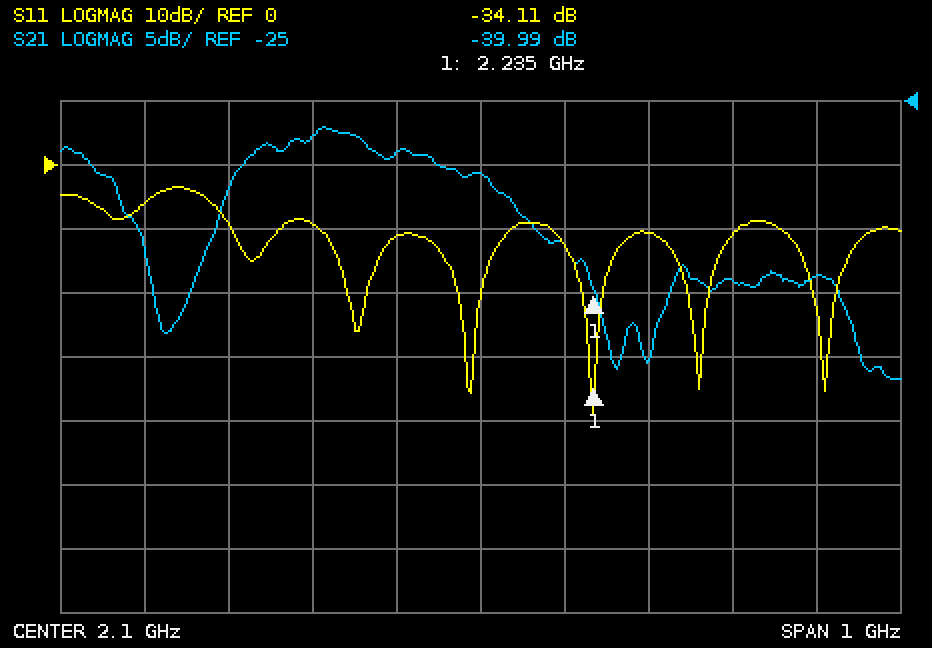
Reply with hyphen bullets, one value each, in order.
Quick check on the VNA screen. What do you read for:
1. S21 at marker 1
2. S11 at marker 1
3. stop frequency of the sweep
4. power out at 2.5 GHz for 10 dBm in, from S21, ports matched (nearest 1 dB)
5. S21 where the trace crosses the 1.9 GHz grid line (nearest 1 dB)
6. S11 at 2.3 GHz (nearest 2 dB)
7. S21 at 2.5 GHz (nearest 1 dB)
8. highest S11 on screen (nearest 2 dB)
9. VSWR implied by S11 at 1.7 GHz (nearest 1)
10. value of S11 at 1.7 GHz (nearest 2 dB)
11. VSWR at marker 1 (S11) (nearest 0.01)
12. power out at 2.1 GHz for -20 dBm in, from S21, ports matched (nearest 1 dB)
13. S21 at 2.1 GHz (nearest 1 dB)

- -39.99 dB
- -34.11 dB
- 2.6 GHz
- -29 dBm
- -28 dB
- -10 dB
- -39 dB
- -4 dB
- 3
- -6 dB
- 1.04
- -51 dBm
- -31 dB
